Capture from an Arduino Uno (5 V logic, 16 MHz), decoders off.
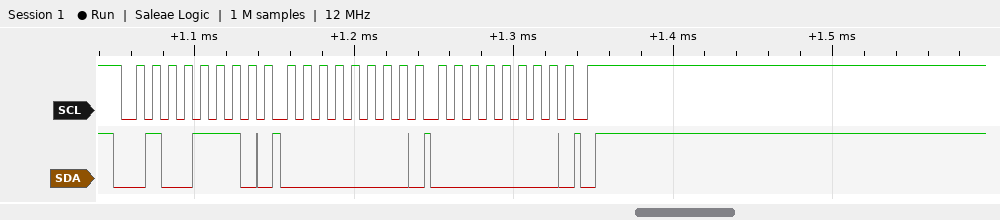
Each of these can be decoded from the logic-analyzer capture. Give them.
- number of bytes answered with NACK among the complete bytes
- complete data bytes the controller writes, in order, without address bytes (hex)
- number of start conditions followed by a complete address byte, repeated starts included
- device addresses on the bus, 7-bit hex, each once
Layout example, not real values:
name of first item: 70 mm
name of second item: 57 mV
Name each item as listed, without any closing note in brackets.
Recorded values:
number of bytes answered with NACK among the complete bytes: 0
complete data bytes the controller writes, in order, without address bytes: 00 00
number of start conditions followed by a complete address byte, repeated starts included: 1
device addresses on the bus, 7-bit hex, each once: 0x27
